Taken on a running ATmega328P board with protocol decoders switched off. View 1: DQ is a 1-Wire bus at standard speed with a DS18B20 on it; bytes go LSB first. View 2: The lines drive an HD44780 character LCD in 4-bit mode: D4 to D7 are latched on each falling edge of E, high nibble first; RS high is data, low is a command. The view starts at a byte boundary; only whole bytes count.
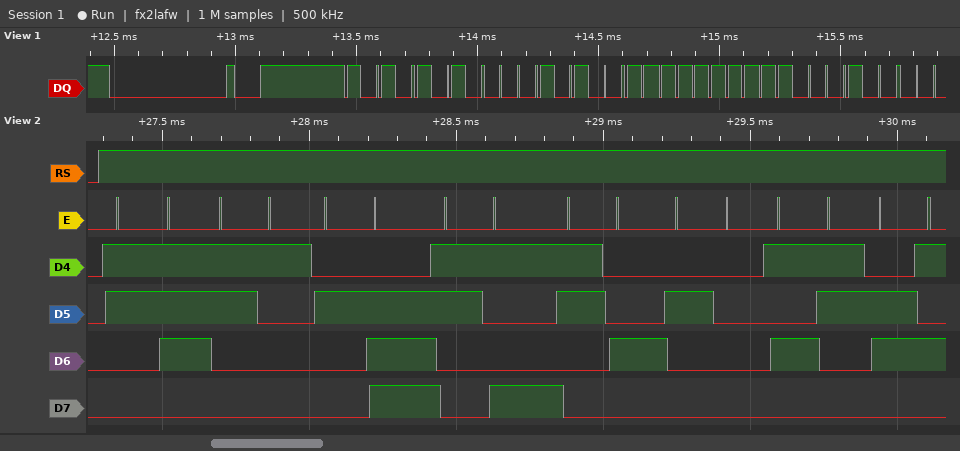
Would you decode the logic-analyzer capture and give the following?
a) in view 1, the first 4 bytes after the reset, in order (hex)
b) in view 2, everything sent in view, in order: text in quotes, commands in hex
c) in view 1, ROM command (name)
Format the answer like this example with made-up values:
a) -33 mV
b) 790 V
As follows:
a) 55 28 FF 23
b) "71.94 Se"
c) Match ROM
